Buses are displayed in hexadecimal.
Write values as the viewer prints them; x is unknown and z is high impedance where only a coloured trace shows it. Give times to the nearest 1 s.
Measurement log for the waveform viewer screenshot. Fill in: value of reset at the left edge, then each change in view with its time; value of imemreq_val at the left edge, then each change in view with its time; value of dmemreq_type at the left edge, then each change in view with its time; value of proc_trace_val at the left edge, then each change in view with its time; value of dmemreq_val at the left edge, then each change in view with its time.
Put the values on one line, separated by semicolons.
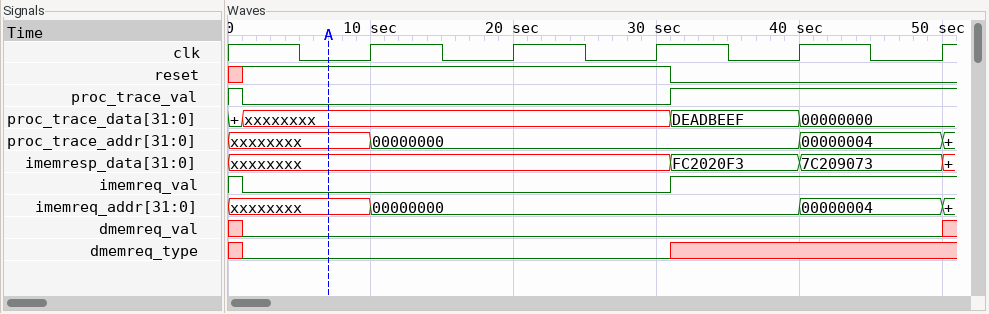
x, 1 at 1 s, 0 at 31 s; 1, 0 at 1 s, 1 at 31 s; x, 0 at 1 s, x at 31 s; 1, 0 at 1 s, 1 at 31 s; x, 0 at 1 s, x at 50 s
